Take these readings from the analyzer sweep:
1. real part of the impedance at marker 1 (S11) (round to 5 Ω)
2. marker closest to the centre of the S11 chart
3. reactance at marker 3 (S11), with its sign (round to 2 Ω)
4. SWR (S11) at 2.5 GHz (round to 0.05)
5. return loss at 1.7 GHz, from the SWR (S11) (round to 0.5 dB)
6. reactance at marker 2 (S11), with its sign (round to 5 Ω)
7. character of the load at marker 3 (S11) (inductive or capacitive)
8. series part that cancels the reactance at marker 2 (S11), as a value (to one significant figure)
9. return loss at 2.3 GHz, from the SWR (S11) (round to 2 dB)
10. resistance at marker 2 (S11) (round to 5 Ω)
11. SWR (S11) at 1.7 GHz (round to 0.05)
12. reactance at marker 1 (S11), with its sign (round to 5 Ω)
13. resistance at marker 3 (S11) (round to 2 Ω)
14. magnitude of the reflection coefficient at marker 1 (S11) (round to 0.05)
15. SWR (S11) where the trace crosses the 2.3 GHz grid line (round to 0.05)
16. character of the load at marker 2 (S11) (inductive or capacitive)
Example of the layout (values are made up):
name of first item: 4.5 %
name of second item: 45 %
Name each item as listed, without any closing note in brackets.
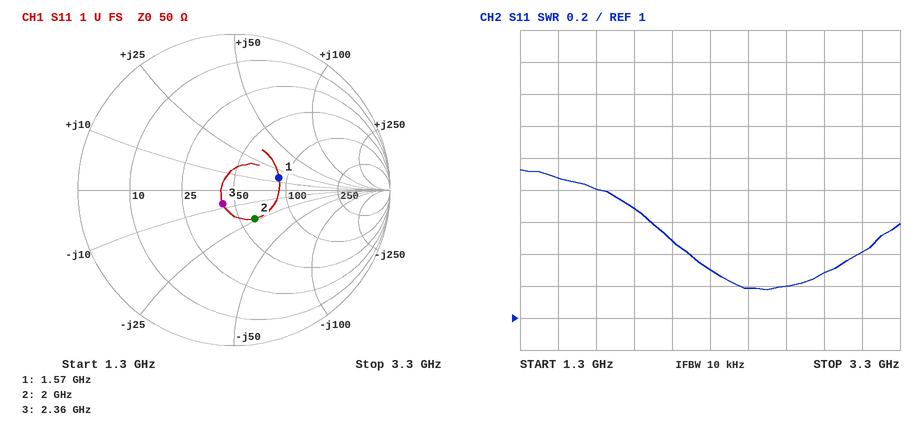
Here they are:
real part of the impedance at marker 1 (S11): 90 Ω
marker closest to the centre of the S11 chart: marker 3
reactance at marker 3 (S11), with its sign: -8 Ω
SWR (S11) at 2.5 GHz: 1.20
return loss at 1.7 GHz, from the SWR (S11): 11.0 dB
reactance at marker 2 (S11), with its sign: -25 Ω
character of the load at marker 3 (S11): capacitive
series part that cancels the reactance at marker 2 (S11), as a value: 2 nH
return loss at 2.3 GHz, from the SWR (S11): 18 dB
resistance at marker 2 (S11): 60 Ω
SWR (S11) at 1.7 GHz: 1.80
reactance at marker 1 (S11), with its sign: +15 Ω
resistance at marker 3 (S11): 42 Ω
magnitude of the reflection coefficient at marker 1 (S11): 0.30
SWR (S11) where the trace crosses the 2.3 GHz grid line: 1.30
character of the load at marker 2 (S11): capacitive
